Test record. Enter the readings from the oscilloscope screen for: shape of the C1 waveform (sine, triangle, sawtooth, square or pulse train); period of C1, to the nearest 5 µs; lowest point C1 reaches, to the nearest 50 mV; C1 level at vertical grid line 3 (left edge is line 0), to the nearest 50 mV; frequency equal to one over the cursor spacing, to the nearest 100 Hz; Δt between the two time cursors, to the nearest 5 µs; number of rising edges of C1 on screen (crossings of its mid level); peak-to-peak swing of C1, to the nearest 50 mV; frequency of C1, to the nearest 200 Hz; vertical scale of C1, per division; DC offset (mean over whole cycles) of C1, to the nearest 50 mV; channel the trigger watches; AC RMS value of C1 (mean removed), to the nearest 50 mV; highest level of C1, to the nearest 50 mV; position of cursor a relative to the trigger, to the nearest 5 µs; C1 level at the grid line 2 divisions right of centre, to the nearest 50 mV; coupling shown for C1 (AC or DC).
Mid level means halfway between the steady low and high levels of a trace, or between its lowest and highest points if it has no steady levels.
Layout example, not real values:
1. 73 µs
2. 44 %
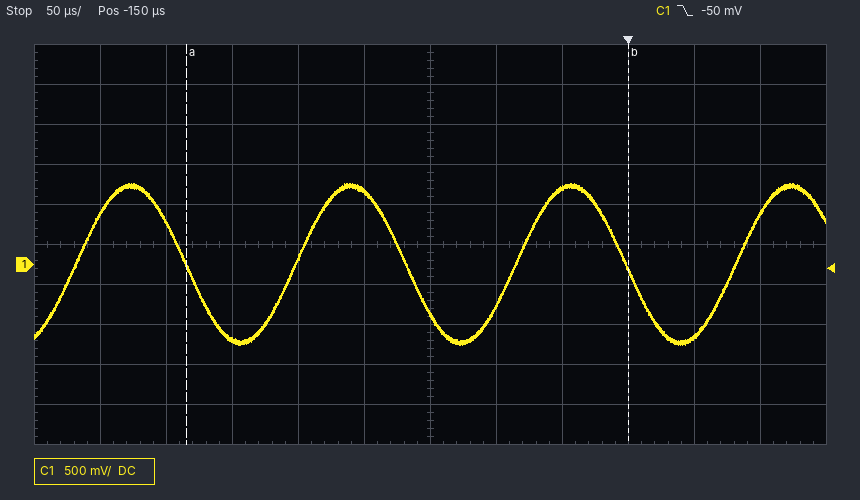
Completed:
1. sine
2. 165 µs
3. -1.00 V
4. -950 mV
5. 3.0 kHz
6. 335 µs
7. 4
8. 2.00 V
9. 6.0 kHz
10. 500 mV
11. 0 mV
12. C1
13. 700 mV
14. 1.00 V
15. -335 µs
16. 950 mV
17. DC
